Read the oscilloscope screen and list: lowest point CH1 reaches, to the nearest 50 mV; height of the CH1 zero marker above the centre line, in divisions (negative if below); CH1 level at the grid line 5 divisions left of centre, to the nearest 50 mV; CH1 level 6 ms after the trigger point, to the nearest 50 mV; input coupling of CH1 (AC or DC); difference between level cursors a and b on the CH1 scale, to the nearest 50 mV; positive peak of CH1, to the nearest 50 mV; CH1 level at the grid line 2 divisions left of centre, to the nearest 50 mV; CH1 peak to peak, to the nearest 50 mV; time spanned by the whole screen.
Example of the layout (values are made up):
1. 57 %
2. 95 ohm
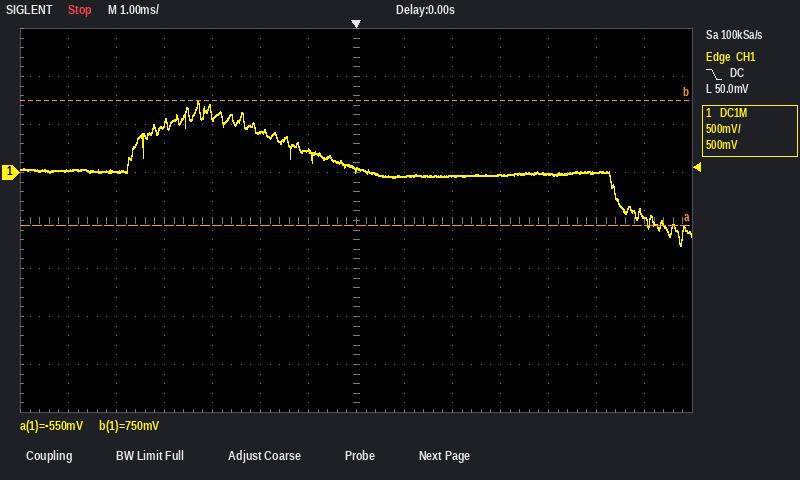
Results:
1. -750 mV
2. +1.0 div
3. 0 mV
4. -450 mV
5. DC
6. 1.30 V
7. 750 mV
8. 400 mV
9. 1.50 V
10. 14 ms
